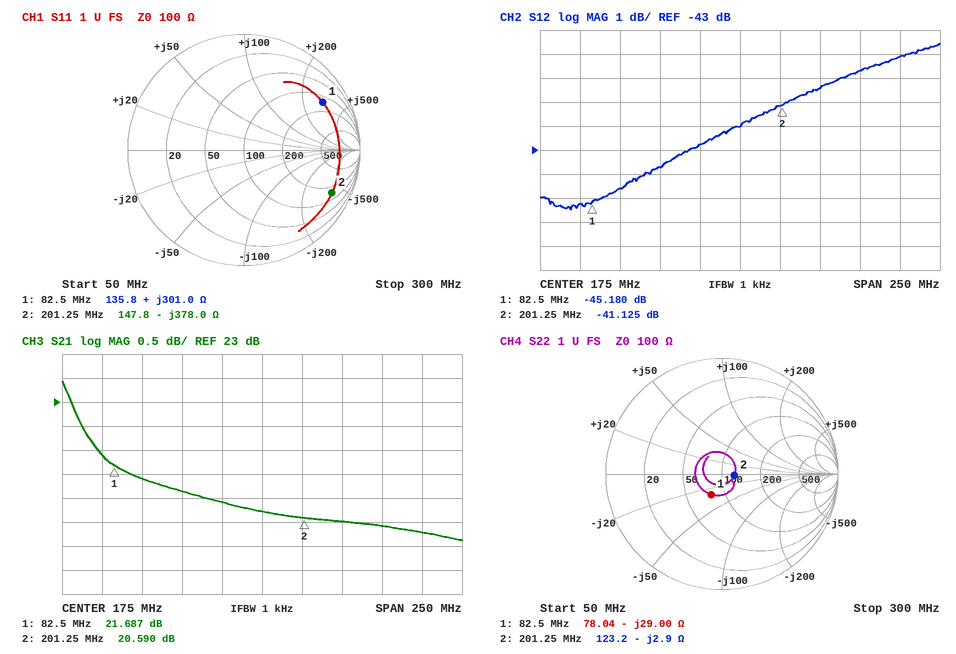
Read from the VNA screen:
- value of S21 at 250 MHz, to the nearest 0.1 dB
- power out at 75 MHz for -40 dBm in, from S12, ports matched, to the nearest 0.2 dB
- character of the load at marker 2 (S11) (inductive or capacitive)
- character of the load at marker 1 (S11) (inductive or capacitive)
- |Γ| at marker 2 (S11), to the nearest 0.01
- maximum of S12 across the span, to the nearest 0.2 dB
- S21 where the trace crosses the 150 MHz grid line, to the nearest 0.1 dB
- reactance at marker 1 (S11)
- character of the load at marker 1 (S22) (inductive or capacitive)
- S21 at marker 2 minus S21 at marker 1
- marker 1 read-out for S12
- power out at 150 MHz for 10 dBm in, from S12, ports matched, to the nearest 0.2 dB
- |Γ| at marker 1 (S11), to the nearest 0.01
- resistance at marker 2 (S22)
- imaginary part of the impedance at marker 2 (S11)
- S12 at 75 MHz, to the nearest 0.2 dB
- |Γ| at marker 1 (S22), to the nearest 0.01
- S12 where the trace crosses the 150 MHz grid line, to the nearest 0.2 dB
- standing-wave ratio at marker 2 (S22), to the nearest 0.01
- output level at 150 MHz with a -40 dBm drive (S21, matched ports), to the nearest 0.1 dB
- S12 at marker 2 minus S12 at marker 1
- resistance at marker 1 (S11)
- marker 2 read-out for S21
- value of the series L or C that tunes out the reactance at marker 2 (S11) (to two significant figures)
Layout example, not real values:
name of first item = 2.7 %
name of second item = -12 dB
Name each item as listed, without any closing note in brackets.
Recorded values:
value of S21 at 250 MHz, to the nearest 0.1 dB = 20.4 dB
power out at 75 MHz for -40 dBm in, from S12, ports matched, to the nearest 0.2 dB = -85.2 dBm
character of the load at marker 2 (S11) = capacitive
character of the load at marker 1 (S11) = inductive
|Γ| at marker 2 (S11), to the nearest 0.01 = 0.84
maximum of S12 across the span, to the nearest 0.2 dB = -38.6 dB
S21 where the trace crosses the 150 MHz grid line, to the nearest 0.1 dB = 20.9 dB
reactance at marker 1 = +301.0 Ω
character of the load at marker 1 (S22) = capacitive
S21 at marker 2 minus S21 at marker 1 = -1.097 dB
marker 1 read-out for S12 = -45.180 dB
power out at 150 MHz for 10 dBm in, from S12, ports matched, to the nearest 0.2 dB = -32.8 dBm
|Γ| at marker 1 (S11), to the nearest 0.01 = 0.79
resistance at marker 2 = 123.2 Ω
imaginary part of the impedance at marker 2 = -378.0 Ω
S12 at 75 MHz, to the nearest 0.2 dB = -45.2 dB
|Γ| at marker 1 (S22), to the nearest 0.01 = 0.20
S12 where the trace crosses the 150 MHz grid line, to the nearest 0.2 dB = -42.8 dB
standing-wave ratio at marker 2 (S22), to the nearest 0.01 = 1.23
output level at 150 MHz with a -40 dBm drive (S21, matched ports), to the nearest 0.1 dB = -19.1 dBm
S12 at marker 2 minus S12 at marker 1 = 4.055 dB
resistance at marker 1 = 135.8 Ω
marker 2 read-out for S21 = 20.590 dB
value of the series L or C that tunes out the reactance at marker 2 (S11) = 300 nH
